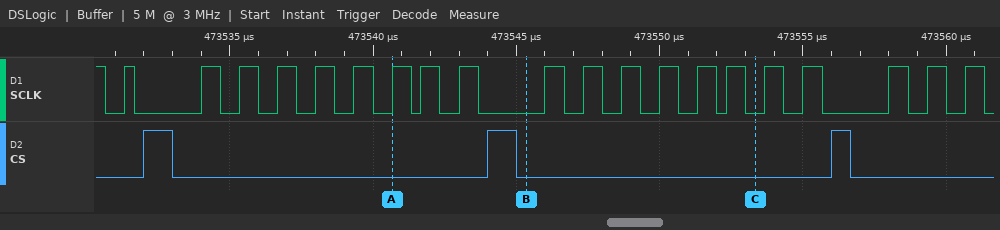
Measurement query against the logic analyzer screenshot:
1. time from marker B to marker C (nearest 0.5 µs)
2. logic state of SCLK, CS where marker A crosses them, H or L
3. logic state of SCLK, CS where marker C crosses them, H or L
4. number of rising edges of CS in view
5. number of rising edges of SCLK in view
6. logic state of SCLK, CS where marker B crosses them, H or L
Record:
8 µs
SCLK=H, CS=L
SCLK=L, CS=L
3
20
SCLK=L, CS=L
